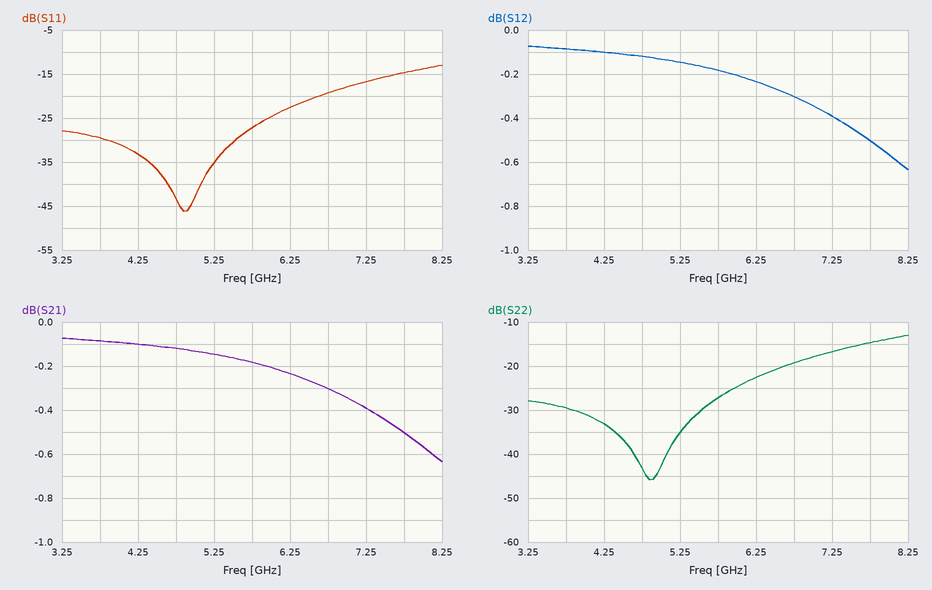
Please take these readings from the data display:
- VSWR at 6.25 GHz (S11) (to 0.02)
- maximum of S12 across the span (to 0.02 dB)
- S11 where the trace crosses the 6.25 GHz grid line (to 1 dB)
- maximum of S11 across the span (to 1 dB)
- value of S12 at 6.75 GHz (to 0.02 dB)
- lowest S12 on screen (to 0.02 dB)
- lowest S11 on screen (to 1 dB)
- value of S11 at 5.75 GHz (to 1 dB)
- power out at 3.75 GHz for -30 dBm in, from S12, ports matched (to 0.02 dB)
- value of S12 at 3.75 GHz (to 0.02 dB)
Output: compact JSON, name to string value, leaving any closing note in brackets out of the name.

{"VSWR at 6.25 GHz (S11)": "1.16", "maximum of S12 across the span": "-0.08 dB", "S11 where the trace crosses the 6.25 GHz grid line": "-23 dB", "maximum of S11 across the span": "-13 dB", "value of S12 at 6.75 GHz": "-0.30 dB", "lowest S12 on screen": "-0.64 dB", "lowest S11 on screen": "-46 dB", "value of S11 at 5.75 GHz": "-27 dB", "power out at 3.75 GHz for -30 dBm in, from S12, ports matched": "-30.08 dBm", "value of S12 at 3.75 GHz": "-0.08 dB"}
